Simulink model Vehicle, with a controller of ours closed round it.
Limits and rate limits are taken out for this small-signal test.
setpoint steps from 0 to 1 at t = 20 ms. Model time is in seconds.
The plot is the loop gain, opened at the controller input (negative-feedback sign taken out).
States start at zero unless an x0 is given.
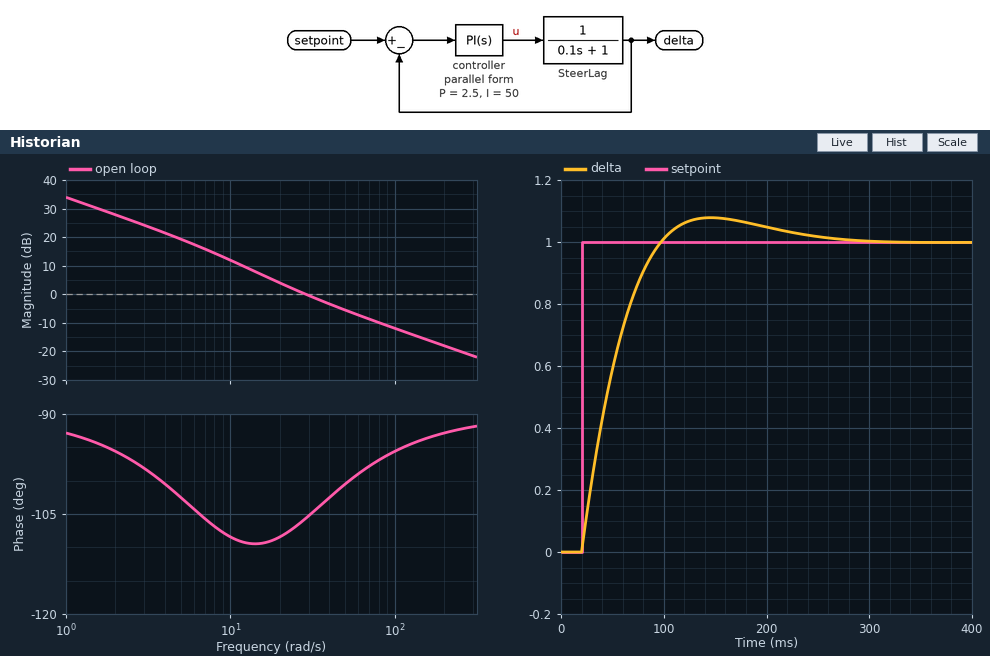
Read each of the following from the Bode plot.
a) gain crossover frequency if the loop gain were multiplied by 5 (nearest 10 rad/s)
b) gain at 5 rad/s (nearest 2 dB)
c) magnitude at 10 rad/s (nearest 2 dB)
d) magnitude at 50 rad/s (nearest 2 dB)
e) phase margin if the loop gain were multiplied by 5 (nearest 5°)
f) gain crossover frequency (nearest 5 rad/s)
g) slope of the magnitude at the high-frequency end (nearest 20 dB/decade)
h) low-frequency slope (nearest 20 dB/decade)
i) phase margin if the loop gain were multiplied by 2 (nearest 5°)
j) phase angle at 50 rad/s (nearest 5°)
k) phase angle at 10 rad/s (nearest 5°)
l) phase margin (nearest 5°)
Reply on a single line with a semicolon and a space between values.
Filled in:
130 rad/s; 20 dB; 12 dB; -6 dB; 85°; 30 rad/s; -20 dB/decade; -20 dB/decade; 80°; -100°; -110°; 75°
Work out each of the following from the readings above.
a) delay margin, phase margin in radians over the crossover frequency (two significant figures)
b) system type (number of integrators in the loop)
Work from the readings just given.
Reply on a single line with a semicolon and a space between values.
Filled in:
0.044 s; 1
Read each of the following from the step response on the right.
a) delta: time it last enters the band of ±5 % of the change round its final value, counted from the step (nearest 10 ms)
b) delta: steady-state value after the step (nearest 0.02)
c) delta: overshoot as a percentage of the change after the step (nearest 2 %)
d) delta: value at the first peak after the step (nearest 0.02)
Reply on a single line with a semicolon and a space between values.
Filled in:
180 ms; 1.00; 8 %; 1.08
